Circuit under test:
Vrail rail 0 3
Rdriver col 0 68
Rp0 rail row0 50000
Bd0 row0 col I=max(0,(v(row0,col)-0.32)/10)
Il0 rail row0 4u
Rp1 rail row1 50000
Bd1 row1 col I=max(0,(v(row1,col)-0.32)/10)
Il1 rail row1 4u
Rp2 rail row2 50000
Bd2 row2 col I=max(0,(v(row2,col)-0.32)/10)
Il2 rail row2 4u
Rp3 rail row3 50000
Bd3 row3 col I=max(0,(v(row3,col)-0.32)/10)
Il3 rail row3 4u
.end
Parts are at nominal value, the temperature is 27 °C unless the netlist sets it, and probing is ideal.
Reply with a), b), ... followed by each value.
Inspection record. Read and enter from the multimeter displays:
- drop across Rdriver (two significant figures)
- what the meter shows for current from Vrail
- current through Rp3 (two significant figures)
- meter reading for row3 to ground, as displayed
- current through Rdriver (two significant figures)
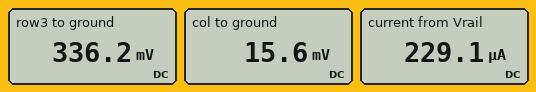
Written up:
a) 16 mV
b) 229.1 µA
c) 53 µA
d) 336.2 mV
e) 230 µA
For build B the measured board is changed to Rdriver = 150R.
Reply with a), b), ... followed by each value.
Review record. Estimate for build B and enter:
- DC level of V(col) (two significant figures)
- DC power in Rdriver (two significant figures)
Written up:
a) 34 mV
b) 7.8 µW
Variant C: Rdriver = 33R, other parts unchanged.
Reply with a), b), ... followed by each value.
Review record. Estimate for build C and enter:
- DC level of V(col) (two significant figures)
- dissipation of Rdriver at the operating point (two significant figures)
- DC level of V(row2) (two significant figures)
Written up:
a) 7.6 mV
b) 1.7 µW
c) 330 mV
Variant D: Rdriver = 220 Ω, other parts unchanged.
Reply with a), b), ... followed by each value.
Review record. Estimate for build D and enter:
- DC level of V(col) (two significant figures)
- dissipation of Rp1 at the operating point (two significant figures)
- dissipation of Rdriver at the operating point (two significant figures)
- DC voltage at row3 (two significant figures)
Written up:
a) 50 mV
b) 140 µW
c) 11 µW
d) 370 mV
